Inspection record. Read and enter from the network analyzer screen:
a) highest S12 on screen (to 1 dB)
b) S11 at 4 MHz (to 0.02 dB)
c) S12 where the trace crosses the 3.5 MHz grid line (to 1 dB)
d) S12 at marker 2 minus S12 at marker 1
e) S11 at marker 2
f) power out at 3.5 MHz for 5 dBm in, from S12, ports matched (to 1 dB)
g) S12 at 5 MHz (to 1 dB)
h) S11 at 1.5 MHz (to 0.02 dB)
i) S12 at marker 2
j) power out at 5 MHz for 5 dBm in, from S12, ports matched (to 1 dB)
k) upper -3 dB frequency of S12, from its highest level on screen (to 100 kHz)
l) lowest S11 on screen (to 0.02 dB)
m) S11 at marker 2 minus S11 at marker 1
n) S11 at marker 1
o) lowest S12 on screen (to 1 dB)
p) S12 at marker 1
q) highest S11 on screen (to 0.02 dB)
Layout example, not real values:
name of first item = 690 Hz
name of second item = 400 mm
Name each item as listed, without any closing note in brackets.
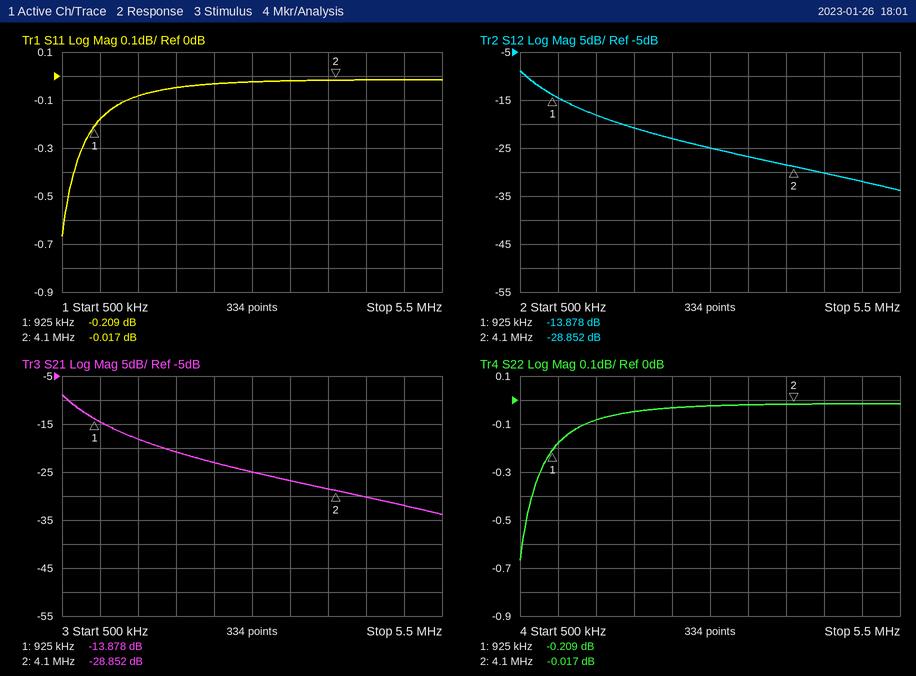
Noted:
highest S12 on screen = -9 dB
S11 at 4 MHz = -0.02 dB
S12 where the trace crosses the 3.5 MHz grid line = -27 dB
S12 at marker 2 minus S12 at marker 1 = -14.974 dB
S11 at marker 2 = -0.017 dB
power out at 3.5 MHz for 5 dBm in, from S12, ports matched = -22 dBm
S12 at 5 MHz = -32 dB
S11 at 1.5 MHz = -0.08 dB
S12 at marker 2 = -28.852 dB
power out at 5 MHz for 5 dBm in, from S12, ports matched = -27 dBm
upper -3 dB frequency of S12, from its highest level on screen = 700 kHz
lowest S11 on screen = -0.66 dB
S11 at marker 2 minus S11 at marker 1 = 0.192 dB
S11 at marker 1 = -0.209 dB
lowest S12 on screen = -34 dB
S12 at marker 1 = -13.878 dB
highest S11 on screen = -0.02 dB
